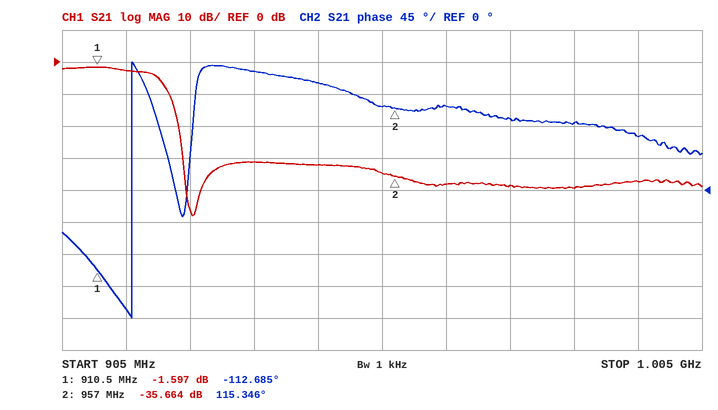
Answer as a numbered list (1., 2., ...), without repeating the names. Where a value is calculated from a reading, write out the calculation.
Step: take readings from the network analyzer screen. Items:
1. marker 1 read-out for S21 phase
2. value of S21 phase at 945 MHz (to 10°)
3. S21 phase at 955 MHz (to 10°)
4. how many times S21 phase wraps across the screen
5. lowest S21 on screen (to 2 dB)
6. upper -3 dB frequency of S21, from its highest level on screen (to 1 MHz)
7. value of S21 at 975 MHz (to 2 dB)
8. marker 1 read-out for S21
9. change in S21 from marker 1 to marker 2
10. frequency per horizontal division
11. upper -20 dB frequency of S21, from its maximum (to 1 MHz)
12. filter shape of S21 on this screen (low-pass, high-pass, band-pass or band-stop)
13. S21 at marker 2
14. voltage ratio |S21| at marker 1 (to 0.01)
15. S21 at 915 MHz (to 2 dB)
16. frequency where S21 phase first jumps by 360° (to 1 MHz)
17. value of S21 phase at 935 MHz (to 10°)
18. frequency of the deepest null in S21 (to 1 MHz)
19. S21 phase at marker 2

1. -112.685°
2. 150°
3. 120°
4. 1
5. -48 dB
6. 920 MHz
7. -38 dB
8. -1.597 dB
9. -35.664 − (-1.597) = -34.067 dB
10. 10 MHz
11. 923 MHz
12. low-pass
13. -35.664 dB
14. 10^(-1.597/20) ≈ 0.83
15. -2 dB
16. 916 MHz
17. 170°
18. 925 MHz
19. 115.346°
